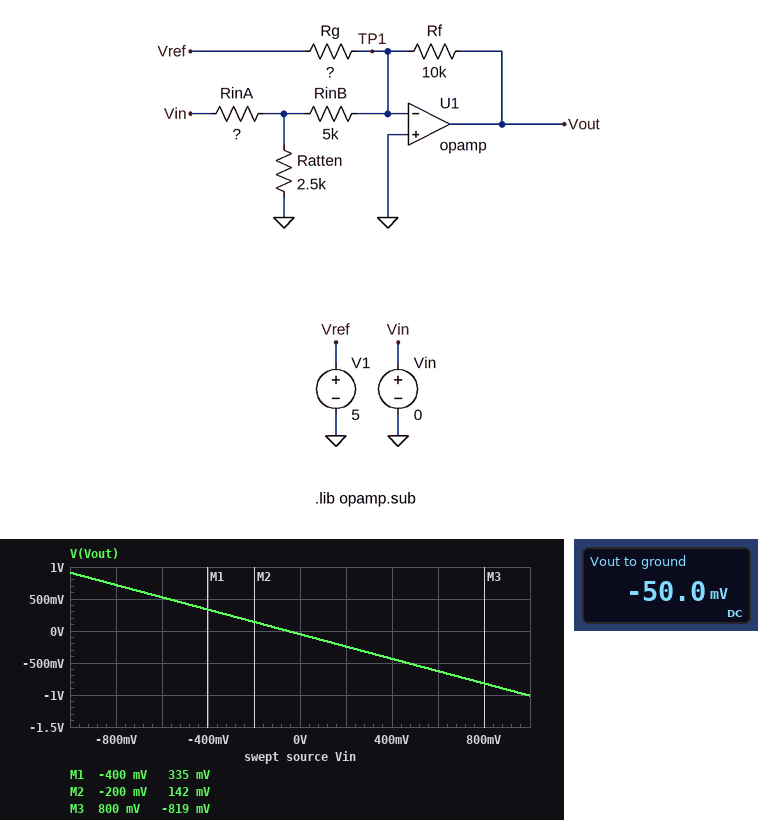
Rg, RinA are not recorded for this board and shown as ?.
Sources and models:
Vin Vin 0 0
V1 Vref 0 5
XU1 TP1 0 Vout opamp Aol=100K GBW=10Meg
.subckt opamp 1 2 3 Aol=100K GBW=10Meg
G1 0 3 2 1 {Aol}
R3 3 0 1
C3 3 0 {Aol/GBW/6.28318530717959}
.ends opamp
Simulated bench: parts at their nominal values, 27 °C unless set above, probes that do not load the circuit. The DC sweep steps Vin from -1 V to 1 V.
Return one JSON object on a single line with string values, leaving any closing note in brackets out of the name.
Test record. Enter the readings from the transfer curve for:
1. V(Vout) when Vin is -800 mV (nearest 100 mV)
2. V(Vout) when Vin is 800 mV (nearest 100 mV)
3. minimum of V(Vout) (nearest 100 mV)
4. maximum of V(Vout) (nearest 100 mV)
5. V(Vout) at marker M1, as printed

{"V(Vout) when Vin is -800 mV": "700 mV", "V(Vout) when Vin is 800 mV": "-800 mV", "minimum of V(Vout)": "-1.0 V", "maximum of V(Vout)": "900 mV", "V(Vout) at marker M1, as printed": "335 mV"}
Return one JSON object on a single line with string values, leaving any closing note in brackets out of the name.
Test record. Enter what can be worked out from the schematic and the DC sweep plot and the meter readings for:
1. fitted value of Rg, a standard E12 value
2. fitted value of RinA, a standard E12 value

{"fitted value of Rg, a standard E12 value": "1 MΩ", "fitted value of RinA, a standard E12 value": "1.8 kΩ"}
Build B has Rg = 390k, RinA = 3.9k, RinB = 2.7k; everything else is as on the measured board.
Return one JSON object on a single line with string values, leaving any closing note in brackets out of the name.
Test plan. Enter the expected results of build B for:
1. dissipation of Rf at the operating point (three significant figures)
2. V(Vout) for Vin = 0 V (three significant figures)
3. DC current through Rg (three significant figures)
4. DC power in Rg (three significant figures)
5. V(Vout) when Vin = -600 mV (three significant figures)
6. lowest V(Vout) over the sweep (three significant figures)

{"dissipation of Rf at the operating point": "1.64 µW", "V(Vout) for Vin = 0 V": "-128 mV", "DC current through Rg": "12.8 µA", "DC power in Rg": "64.1 µW", "V(Vout) when Vin = -600 mV": "427 mV", "lowest V(Vout) over the sweep": "-1.05 V"}
